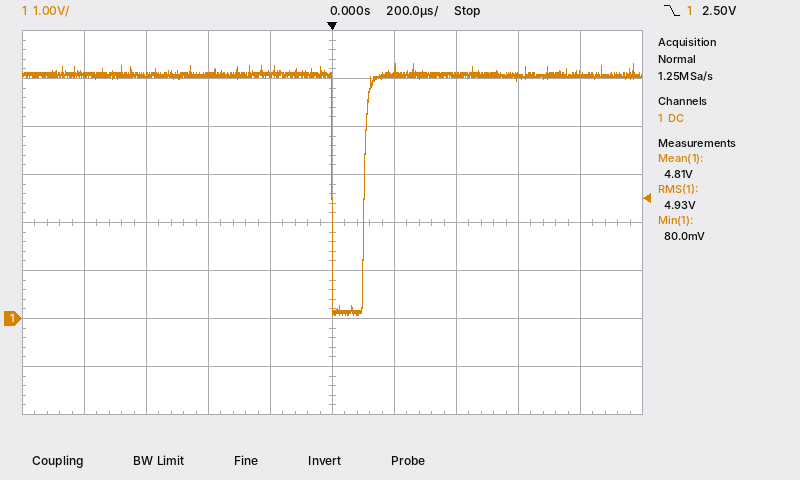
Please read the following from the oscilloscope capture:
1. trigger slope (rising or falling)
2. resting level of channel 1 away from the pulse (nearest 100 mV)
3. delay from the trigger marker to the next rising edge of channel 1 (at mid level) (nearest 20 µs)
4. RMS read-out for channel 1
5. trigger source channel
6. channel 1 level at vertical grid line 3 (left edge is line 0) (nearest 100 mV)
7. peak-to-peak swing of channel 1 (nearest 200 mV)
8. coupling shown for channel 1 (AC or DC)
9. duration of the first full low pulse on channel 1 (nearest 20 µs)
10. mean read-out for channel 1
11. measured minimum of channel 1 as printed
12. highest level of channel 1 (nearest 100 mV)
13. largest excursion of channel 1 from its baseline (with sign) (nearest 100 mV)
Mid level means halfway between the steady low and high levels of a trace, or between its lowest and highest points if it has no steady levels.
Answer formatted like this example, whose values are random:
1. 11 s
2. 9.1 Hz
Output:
1. falling
2. 5.1 V
3. 100 µs
4. 4.93 V
5. channel 1
6. 5.1 V
7. 5.2 V
8. DC
9. 100 µs
10. 4.81 V
11. 80.0 mV
12. 5.3 V
13. -5.0 V
